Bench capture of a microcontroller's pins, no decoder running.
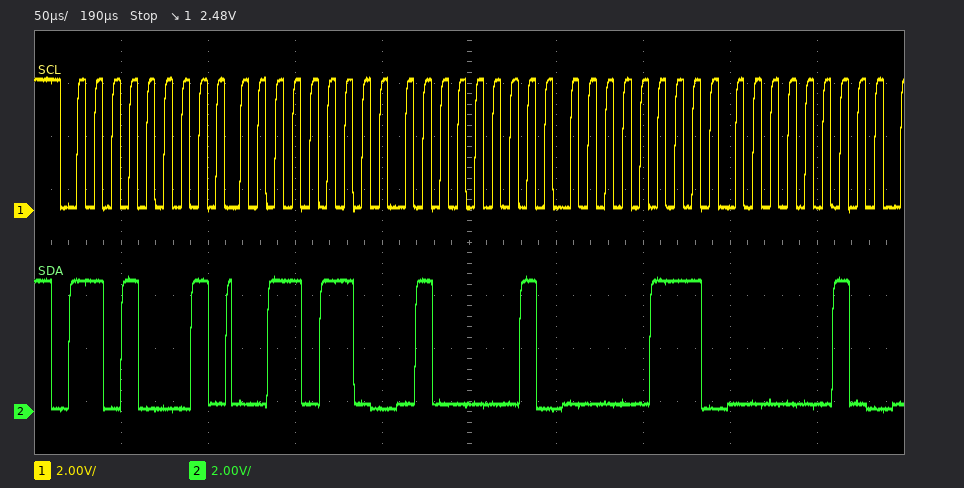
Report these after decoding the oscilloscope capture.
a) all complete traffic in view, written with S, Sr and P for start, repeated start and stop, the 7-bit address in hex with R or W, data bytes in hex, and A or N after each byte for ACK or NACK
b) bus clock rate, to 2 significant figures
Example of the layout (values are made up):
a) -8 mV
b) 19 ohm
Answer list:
a) S 68R A 36 A 41 A 07 A 02 A
b) 100 kHz
